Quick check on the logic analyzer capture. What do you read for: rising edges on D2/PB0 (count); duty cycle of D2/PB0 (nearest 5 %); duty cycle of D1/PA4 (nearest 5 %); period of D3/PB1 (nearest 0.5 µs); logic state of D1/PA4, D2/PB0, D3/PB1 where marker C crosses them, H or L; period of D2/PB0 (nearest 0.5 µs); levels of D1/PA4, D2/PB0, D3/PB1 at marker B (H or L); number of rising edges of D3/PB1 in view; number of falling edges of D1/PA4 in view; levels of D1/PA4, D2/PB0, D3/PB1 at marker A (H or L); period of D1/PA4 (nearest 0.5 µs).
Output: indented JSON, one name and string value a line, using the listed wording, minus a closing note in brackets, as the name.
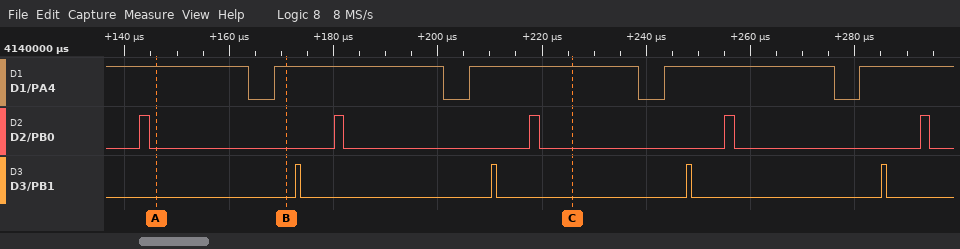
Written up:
{
  "rising edges on D2/PB0": "5",
  "duty cycle of D2/PB0": "5 %",
  "duty cycle of D1/PA4": "85 %",
  "period of D3/PB1": "37.5 µs",
  "logic state of D1/PA4, D2/PB0, D3/PB1 where marker C crosses them, H or L": "D1/PA4=H, D2/PB0=L, D3/PB1=L",
  "period of D2/PB0": "37.5 µs",
  "levels of D1/PA4, D2/PB0, D3/PB1 at marker B": "D1/PA4=H, D2/PB0=L, D3/PB1=L",
  "number of rising edges of D3/PB1 in view": "4",
  "number of falling edges of D1/PA4 in view": "4",
  "levels of D1/PA4, D2/PB0, D3/PB1 at marker A": "D1/PA4=H, D2/PB0=L, D3/PB1=L",
  "period of D1/PA4": "37.5 µs"
}
